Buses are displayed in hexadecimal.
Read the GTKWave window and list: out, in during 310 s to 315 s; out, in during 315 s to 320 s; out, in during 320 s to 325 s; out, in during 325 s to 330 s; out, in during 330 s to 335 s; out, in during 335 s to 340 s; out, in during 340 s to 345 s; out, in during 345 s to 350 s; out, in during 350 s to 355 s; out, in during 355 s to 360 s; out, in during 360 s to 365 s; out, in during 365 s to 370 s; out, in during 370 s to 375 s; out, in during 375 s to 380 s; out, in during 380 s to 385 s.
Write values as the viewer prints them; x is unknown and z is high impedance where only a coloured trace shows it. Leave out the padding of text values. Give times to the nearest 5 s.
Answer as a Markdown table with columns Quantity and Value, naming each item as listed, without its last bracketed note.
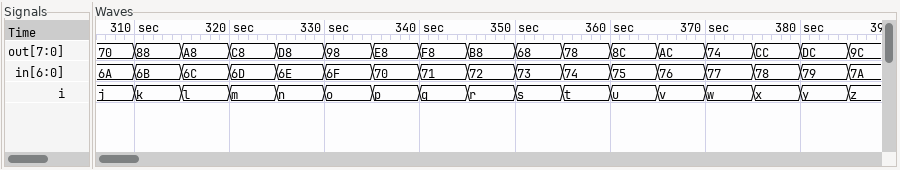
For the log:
| Quantity | Value |
|---|---|
| out, in during 310 s to 315 s | out=88, in=6B |
| out, in during 315 s to 320 s | out=A8, in=6C |
| out, in during 320 s to 325 s | out=C8, in=6D |
| out, in during 325 s to 330 s | out=D8, in=6E |
| out, in during 330 s to 335 s | out=98, in=6F |
| out, in during 335 s to 340 s | out=E8, in=70 |
| out, in during 340 s to 345 s | out=F8, in=71 |
| out, in during 345 s to 350 s | out=B8, in=72 |
| out, in during 350 s to 355 s | out=68, in=73 |
| out, in during 355 s to 360 s | out=78, in=74 |
| out, in during 360 s to 365 s | out=8C, in=75 |
| out, in during 365 s to 370 s | out=AC, in=76 |
| out, in during 370 s to 375 s | out=74, in=77 |
| out, in during 375 s to 380 s | out=CC, in=78 |
| out, in during 380 s to 385 s | out=DC, in=79 |
